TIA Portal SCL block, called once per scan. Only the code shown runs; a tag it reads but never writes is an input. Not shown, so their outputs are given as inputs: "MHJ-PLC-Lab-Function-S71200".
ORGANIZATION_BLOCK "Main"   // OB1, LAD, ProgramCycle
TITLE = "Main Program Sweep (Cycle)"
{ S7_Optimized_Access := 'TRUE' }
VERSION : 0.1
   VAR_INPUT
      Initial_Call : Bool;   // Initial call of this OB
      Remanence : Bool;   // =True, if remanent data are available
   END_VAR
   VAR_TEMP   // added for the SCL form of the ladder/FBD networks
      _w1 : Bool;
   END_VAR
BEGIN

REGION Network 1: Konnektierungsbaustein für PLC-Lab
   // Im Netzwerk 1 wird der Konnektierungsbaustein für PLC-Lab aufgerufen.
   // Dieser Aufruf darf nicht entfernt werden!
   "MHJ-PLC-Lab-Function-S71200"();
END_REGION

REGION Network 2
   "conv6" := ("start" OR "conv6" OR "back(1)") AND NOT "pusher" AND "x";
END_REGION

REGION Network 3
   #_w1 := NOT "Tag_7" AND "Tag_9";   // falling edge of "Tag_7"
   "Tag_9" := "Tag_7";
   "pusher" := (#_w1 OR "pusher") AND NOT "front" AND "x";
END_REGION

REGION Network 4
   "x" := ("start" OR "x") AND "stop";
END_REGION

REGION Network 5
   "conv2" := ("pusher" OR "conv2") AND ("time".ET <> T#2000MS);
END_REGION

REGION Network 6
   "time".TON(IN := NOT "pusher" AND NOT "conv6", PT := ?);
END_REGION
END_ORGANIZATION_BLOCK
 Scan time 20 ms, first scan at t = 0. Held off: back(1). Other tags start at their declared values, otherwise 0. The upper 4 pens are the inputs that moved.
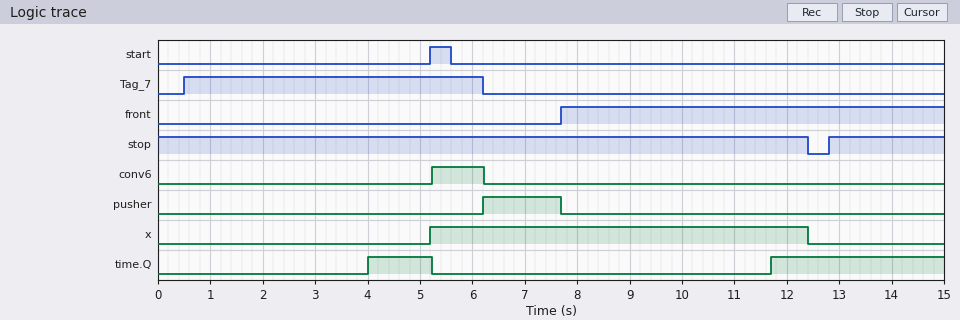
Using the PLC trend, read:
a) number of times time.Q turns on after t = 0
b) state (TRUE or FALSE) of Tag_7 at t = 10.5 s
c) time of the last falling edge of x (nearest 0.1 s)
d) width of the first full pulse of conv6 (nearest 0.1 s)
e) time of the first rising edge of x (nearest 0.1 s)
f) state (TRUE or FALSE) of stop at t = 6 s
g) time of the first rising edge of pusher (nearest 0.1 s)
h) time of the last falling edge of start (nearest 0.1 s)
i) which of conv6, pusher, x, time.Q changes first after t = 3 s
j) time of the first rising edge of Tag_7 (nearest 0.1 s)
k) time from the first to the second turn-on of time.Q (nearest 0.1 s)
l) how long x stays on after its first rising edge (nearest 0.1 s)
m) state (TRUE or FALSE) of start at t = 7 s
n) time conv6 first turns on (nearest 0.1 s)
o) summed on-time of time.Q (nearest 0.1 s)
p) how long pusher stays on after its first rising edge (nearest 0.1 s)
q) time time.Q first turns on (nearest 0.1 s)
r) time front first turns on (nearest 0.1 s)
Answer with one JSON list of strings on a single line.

["2", "FALSE", "12.4 s", "1.0 s", "5.2 s", "TRUE", "6.2 s", "5.6 s", "time.Q", "0.5 s", "7.7 s", "7.2 s", "FALSE", "5.2 s", "4.5 s", "1.5 s", "4.0 s", "7.7 s"]
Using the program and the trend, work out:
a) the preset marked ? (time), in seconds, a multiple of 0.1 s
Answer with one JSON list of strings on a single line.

["4.0 s"]
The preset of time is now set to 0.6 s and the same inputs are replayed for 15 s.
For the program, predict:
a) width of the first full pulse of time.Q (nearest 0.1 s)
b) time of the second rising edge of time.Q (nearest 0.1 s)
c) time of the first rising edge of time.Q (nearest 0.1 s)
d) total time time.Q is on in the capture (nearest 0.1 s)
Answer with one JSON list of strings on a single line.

["4.6 s", "8.3 s", "0.6 s", "11.3 s"]
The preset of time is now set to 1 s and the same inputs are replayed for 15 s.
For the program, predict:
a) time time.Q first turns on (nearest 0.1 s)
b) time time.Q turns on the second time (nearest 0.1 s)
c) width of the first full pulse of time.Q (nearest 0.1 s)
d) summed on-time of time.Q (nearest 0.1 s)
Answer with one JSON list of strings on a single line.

["1.0 s", "8.7 s", "4.2 s", "10.5 s"]
